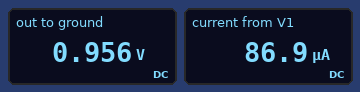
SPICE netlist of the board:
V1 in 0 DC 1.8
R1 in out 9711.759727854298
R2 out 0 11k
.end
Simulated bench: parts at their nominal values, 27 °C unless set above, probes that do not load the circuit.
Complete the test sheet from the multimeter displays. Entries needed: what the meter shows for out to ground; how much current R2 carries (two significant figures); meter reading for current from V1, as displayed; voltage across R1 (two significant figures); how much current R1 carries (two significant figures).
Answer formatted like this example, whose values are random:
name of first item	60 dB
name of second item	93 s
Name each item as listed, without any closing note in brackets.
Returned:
what the meter shows for out to ground	0.956 V
how much current R2 carries	87 µA
meter reading for current from V1, as displayed	86.9 µA
voltage across R1	840 mV
how much current R1 carries	87 µA
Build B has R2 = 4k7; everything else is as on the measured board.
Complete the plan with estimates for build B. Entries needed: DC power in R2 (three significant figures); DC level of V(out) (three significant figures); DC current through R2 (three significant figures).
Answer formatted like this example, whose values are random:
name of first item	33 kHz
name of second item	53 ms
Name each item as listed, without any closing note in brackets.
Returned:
DC power in R2	73.3 µW
DC level of V(out)	587 mV
DC current through R2	125 µA
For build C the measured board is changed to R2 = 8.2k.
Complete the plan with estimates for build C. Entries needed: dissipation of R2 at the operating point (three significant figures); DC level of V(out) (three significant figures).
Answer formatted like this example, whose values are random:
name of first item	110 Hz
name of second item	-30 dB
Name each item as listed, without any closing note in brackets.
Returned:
dissipation of R2 at the operating point	82.8 µW
DC level of V(out)	824 mV
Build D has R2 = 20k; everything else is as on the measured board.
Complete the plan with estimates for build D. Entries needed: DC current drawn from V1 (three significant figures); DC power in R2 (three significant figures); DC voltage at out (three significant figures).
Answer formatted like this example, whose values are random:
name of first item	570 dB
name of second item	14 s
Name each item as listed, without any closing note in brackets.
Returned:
DC current drawn from V1	60.6 µA
DC power in R2	73.4 µW
DC voltage at out	1.21 V
